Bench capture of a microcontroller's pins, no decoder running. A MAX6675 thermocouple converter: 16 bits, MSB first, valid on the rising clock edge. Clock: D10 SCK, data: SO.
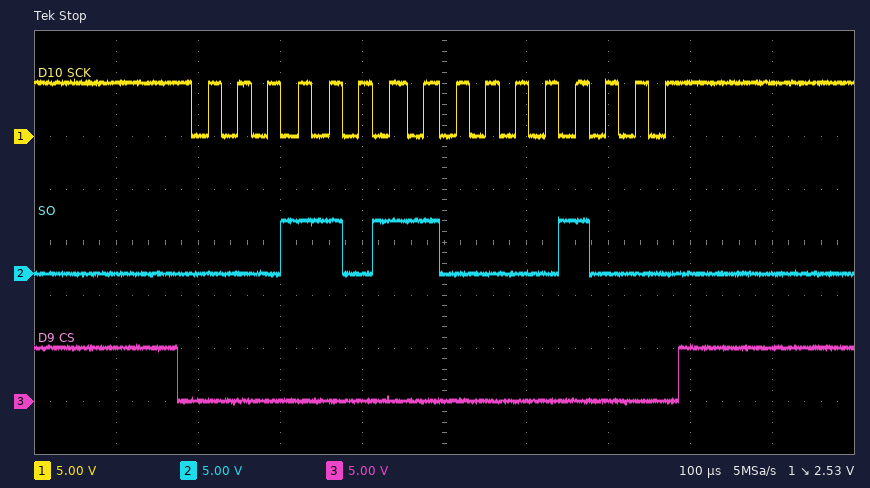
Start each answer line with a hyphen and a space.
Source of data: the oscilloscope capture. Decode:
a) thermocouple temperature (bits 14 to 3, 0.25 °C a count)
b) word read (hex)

- 216.25 °C
- 0x1B08
